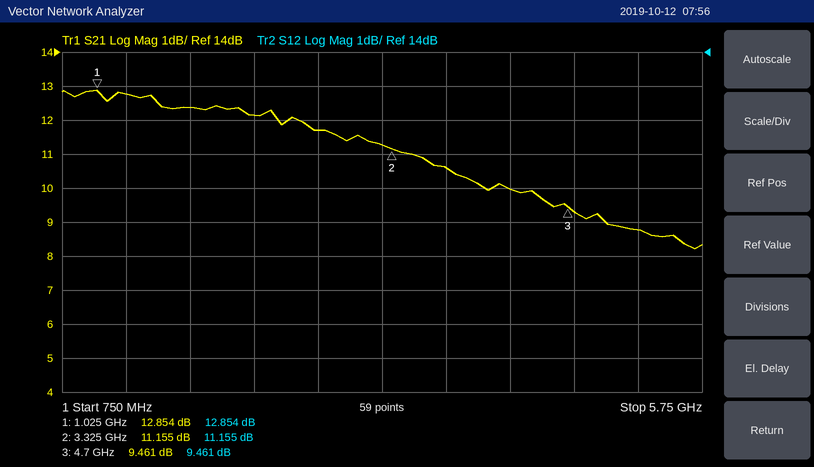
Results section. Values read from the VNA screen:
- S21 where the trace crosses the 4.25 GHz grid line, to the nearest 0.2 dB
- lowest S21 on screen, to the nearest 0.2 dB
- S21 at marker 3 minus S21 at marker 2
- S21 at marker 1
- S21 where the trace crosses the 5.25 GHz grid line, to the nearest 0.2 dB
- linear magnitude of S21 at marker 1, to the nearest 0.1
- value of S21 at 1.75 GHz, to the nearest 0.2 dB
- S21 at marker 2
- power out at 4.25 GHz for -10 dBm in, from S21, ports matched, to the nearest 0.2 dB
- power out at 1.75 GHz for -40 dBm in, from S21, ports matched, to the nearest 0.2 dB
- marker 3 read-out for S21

10.0 dB
8.2 dB
-1.694 dB
12.854 dB
8.8 dB
4.4
12.4 dB
11.155 dB
0.0 dBm
-27.6 dBm
9.461 dB
